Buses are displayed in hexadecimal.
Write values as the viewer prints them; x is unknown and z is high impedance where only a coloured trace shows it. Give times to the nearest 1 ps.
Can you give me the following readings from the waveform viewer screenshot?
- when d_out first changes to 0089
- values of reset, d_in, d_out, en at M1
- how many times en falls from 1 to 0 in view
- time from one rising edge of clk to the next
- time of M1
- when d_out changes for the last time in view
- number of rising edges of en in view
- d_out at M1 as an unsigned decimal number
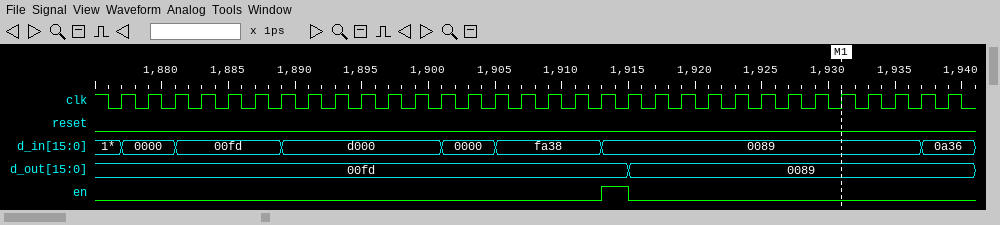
1915 ps
reset=0, d_in=0089, d_out=0089, en=0
1
2 ps
1931 ps
1915 ps
1
137
